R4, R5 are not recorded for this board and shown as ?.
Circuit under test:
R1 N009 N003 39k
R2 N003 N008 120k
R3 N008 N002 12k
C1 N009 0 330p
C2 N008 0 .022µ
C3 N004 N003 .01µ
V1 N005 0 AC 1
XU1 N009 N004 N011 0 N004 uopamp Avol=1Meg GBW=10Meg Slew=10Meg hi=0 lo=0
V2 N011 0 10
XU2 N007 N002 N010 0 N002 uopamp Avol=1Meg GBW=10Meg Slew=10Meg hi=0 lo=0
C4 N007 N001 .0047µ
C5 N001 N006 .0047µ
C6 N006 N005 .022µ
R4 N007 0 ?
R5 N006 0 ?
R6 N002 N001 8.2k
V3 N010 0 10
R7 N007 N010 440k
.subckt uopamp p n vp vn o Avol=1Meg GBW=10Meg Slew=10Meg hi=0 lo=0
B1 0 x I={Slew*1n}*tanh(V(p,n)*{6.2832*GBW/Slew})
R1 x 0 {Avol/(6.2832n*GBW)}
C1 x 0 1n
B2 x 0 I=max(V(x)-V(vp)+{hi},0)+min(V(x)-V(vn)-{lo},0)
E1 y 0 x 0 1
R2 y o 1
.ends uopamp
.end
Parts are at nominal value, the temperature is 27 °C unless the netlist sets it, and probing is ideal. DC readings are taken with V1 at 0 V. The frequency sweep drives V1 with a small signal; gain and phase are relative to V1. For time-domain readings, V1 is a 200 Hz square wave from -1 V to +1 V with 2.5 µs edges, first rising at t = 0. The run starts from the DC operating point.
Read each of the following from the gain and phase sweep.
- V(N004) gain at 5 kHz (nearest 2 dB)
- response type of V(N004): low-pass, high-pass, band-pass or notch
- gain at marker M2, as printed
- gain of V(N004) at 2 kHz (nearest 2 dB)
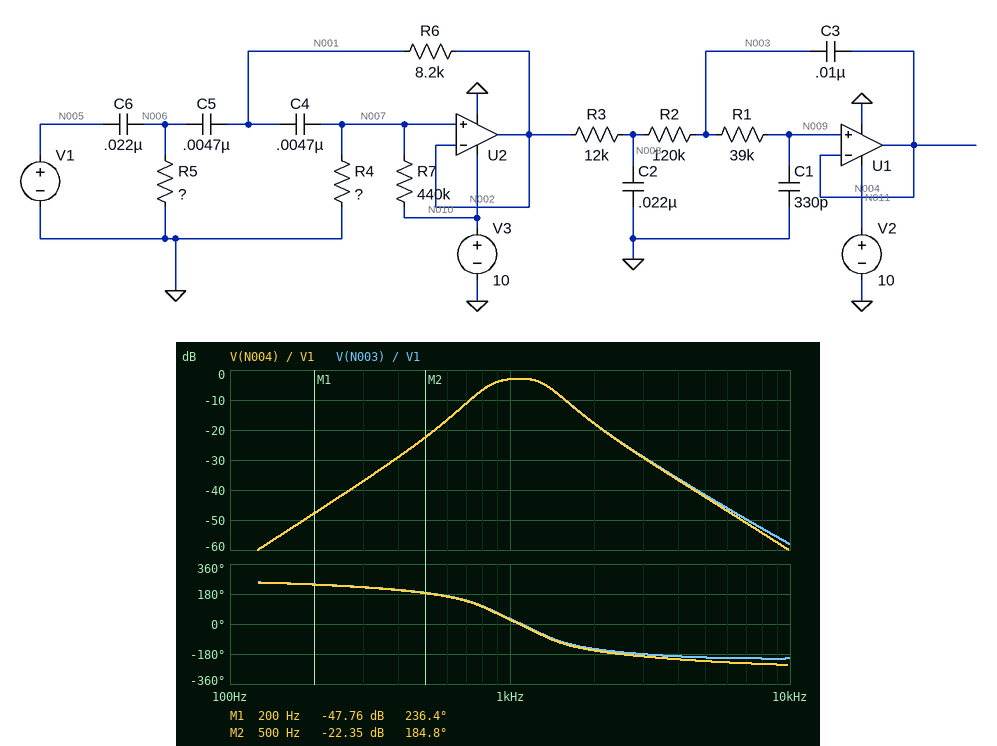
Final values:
-42 dB
band-pass
-22.35 dB
-18 dB
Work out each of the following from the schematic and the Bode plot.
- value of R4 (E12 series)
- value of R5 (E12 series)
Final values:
330 kΩ
2.7 kΩ
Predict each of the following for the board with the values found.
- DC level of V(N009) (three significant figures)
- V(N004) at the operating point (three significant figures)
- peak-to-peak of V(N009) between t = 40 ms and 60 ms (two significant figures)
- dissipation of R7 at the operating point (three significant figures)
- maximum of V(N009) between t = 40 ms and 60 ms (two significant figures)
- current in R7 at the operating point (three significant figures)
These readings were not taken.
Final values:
4.29 V
4.29 V
670 mV
74.2 µW
4.6 V
13.0 µA
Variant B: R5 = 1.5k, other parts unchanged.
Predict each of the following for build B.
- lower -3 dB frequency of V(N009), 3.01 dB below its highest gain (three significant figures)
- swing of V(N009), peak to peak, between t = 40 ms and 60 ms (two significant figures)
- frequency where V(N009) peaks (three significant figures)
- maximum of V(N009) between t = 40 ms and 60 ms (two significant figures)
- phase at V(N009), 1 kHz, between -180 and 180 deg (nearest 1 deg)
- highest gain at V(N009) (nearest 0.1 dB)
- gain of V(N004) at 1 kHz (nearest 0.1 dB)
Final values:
814 Hz
400 mV
1.08 kHz
4.5 V
32 deg
-7.4 dB
-7.5 dB
